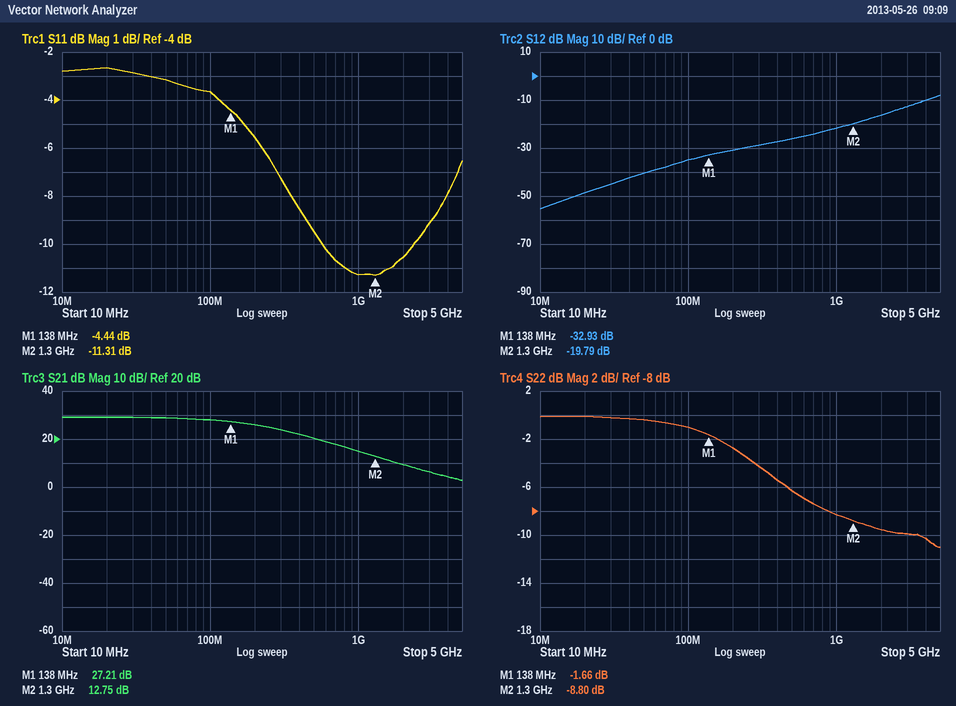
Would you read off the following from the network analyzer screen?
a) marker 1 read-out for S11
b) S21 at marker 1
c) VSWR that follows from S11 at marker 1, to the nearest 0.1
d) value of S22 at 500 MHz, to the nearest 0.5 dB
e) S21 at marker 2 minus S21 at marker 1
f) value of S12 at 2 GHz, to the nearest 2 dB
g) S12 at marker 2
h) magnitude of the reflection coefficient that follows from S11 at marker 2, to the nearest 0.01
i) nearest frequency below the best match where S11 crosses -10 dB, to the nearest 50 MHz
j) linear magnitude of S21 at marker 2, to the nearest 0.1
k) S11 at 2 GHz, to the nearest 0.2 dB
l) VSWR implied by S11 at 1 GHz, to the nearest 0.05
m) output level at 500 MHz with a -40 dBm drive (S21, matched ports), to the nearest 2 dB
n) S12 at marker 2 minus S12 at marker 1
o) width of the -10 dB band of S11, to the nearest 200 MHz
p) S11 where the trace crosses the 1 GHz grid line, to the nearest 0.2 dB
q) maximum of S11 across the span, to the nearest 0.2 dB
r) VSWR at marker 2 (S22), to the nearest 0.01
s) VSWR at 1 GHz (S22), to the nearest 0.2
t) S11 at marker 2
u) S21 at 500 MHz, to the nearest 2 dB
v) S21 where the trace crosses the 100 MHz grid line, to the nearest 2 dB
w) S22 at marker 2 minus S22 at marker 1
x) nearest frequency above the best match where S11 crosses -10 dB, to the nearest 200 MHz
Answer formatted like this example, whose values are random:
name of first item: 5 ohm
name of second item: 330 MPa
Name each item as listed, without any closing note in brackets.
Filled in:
marker 1 read-out for S11: -4.44 dB
S21 at marker 1: 27.21 dB
VSWR that follows from S11 at marker 1, to the nearest 0.1: 4.0
value of S22 at 500 MHz, to the nearest 0.5 dB: -6.5 dB
S21 at marker 2 minus S21 at marker 1: -14.46 dB
value of S12 at 2 GHz, to the nearest 2 dB: -16 dB
S12 at marker 2: -19.79 dB
magnitude of the reflection coefficient that follows from S11 at marker 2, to the nearest 0.01: 0.27
nearest frequency below the best match where S11 crosses -10 dB, to the nearest 50 MHz: 550 MHz
linear magnitude of S21 at marker 2, to the nearest 0.1: 4.3
S11 at 2 GHz, to the nearest 0.2 dB: -10.6 dB
VSWR implied by S11 at 1 GHz, to the nearest 0.05: 1.75
output level at 500 MHz with a -40 dBm drive (S21, matched ports), to the nearest 2 dB: -20 dBm
S12 at marker 2 minus S12 at marker 1: 13.14 dB
width of the -10 dB band of S11, to the nearest 200 MHz: 1.8 GHz
S11 where the trace crosses the 1 GHz grid line, to the nearest 0.2 dB: -11.2 dB
maximum of S11 across the span, to the nearest 0.2 dB: -2.6 dB
VSWR at marker 2 (S22), to the nearest 0.01: 2.14
VSWR at 1 GHz (S22), to the nearest 0.2: 2.2
S11 at marker 2: -11.31 dB
S21 at 500 MHz, to the nearest 2 dB: 20 dB
S21 where the trace crosses the 100 MHz grid line, to the nearest 2 dB: 28 dB
S22 at marker 2 minus S22 at marker 1: -7.14 dB
nearest frequency above the best match where S11 crosses -10 dB, to the nearest 200 MHz: 2.4 GHz
